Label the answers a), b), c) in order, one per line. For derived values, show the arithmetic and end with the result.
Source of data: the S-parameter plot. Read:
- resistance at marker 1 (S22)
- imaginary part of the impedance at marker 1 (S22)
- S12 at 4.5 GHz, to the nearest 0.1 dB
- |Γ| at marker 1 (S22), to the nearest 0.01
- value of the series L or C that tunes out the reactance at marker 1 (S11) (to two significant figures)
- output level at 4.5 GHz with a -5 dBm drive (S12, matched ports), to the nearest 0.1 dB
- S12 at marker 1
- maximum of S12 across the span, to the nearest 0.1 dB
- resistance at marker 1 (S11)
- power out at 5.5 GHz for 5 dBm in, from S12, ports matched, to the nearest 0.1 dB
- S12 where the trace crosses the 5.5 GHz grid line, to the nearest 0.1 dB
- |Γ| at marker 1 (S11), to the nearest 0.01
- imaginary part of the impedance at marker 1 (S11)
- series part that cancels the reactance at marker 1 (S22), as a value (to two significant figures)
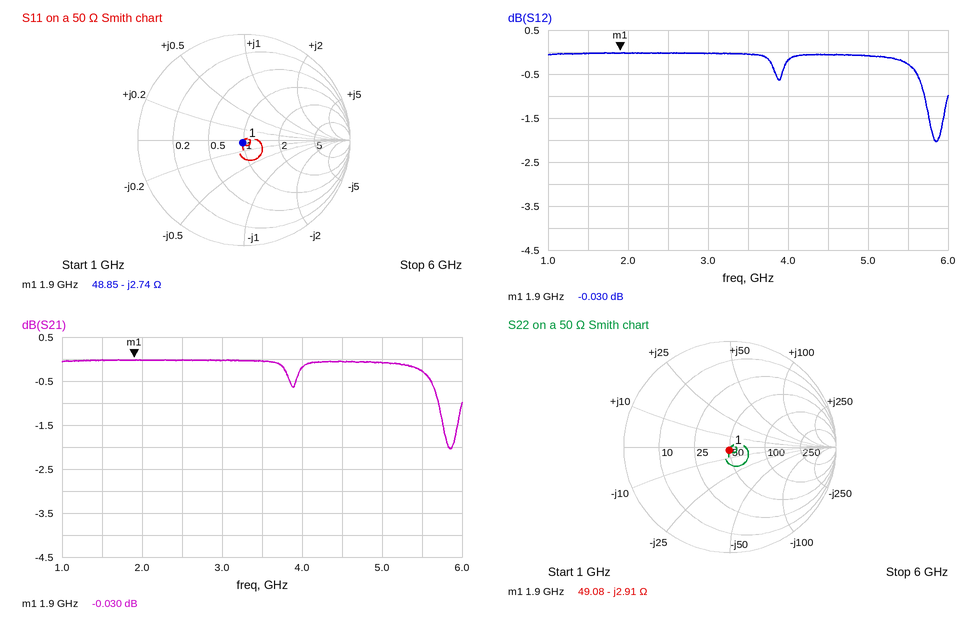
a) 49.08 Ω
b) -2.91 Ω
c) -0.1 dB
d) 0.03
e) L = 2.74 Ω/(2π × 1.9 GHz) ≈ 230 pH
f) -5 dBm + (-0.1 dB) = -5.1 dBm
g) -0.030 dB
h) 0.0 dB
i) 48.85 Ω
j) 5 dBm + (-0.3 dB) = 4.7 dBm
k) -0.3 dB
l) 0.03
m) -2.74 Ω
n) L = 2.91 Ω/(2π × 1.9 GHz) ≈ 244 pH, so 240 pH to two significant figures
